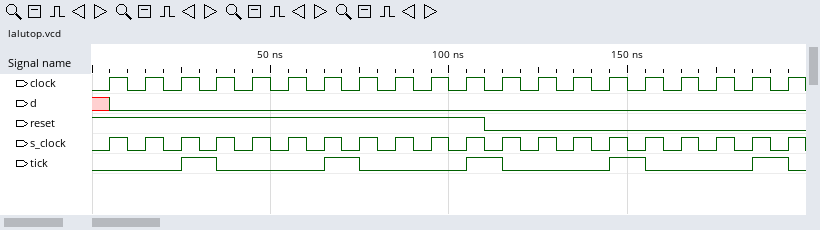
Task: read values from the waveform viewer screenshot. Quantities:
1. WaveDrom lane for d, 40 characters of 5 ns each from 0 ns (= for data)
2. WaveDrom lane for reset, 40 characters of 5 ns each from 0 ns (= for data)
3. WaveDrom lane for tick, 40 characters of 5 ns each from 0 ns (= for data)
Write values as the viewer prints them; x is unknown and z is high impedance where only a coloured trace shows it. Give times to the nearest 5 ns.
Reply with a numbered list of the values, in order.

1. {name: 'd', wave: 'x0......................................'}
2. {name: 'reset', wave: '1.....................0.................'}
3. {name: 'tick', wave: '0....1.0.....1.0.....1.0.....1.0.....1.0'}
